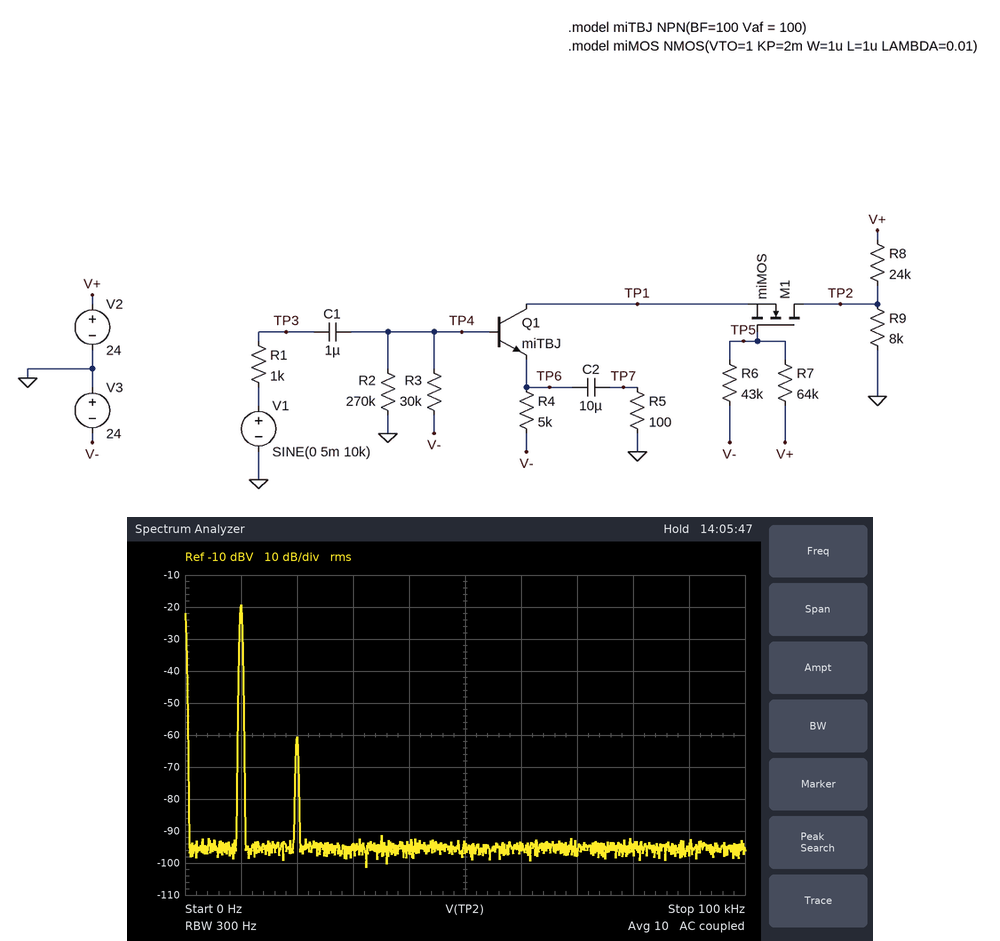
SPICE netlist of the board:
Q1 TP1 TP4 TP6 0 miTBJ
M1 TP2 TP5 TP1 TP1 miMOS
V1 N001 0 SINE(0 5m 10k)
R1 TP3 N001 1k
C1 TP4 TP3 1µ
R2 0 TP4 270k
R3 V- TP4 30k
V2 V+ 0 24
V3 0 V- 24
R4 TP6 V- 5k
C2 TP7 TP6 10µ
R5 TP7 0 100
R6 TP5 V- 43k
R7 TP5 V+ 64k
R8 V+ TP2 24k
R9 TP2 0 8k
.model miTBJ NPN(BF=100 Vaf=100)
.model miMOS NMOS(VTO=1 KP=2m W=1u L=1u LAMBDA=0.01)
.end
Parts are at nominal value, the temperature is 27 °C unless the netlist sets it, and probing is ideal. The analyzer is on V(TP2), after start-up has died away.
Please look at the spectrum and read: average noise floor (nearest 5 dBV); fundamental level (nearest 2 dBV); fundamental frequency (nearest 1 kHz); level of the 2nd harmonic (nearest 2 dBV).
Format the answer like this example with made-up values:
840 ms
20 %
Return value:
-95 dBV
-20 dBV
10 kHz
-60 dBV
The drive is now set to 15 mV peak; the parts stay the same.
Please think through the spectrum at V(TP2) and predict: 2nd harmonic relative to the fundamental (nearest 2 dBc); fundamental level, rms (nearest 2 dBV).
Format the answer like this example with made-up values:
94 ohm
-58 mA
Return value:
-32 dBc
-10 dBV
